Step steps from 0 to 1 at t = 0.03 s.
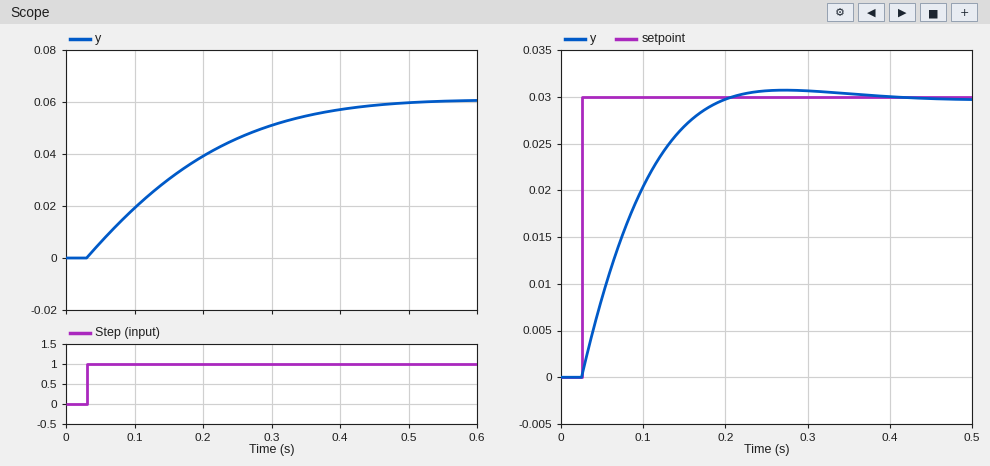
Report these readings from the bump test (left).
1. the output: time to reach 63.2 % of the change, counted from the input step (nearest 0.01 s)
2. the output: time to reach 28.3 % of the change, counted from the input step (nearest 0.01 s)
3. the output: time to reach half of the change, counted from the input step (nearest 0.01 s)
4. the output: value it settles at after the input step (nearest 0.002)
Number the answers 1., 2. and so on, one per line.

1. 0.16 s
2. 0.06 s
3. 0.12 s
4. 0.060
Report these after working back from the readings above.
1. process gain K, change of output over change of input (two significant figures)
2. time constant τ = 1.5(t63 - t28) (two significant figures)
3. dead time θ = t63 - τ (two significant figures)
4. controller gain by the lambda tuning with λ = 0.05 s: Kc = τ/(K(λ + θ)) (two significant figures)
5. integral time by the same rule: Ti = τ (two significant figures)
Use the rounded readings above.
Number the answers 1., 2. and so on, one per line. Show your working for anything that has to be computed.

1. (0.06 - 0) / 1 = 0.060
2. 1.5 × (0.16 - 0.06) = 0.15 s
3. 0.16 - 0.15 = 0.010 s
4. 0.15 / (0.06 × (0.05 + 0.01)) = 42
5. 0.15 s
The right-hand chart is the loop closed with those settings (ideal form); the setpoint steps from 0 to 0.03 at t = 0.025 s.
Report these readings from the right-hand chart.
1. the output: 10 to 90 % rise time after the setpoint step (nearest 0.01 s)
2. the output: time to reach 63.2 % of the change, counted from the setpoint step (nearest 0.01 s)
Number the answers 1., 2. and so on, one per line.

1. 0.12 s
2. 0.07 s
